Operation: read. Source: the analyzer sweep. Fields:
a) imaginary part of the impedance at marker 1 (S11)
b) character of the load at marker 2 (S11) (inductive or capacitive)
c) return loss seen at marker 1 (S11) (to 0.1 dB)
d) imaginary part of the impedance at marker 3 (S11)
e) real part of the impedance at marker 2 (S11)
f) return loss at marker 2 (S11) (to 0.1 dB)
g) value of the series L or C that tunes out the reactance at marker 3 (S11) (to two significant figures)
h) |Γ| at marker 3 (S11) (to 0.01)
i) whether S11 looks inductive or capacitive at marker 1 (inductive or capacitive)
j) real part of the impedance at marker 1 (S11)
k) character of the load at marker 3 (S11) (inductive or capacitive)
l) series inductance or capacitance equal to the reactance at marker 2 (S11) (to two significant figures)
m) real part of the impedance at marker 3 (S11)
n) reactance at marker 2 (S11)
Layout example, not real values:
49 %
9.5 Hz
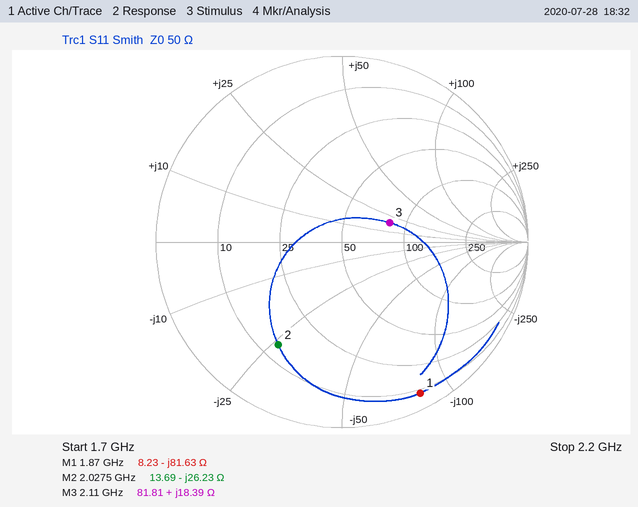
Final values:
-81.63 Ω
capacitive
0.8 dB
+18.39 Ω
13.69 Ω
3.7 dB
4.1 pF
0.28
capacitive
8.23 Ω
inductive
3.0 pF
81.81 Ω
-26.23 Ω
